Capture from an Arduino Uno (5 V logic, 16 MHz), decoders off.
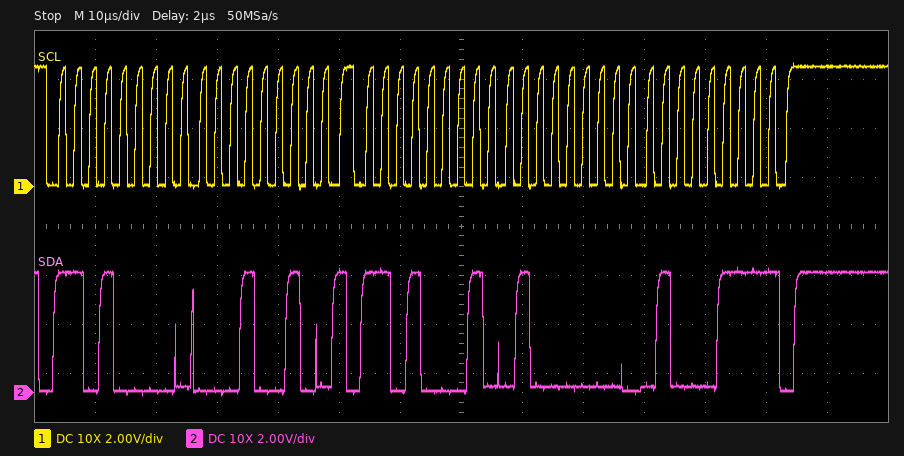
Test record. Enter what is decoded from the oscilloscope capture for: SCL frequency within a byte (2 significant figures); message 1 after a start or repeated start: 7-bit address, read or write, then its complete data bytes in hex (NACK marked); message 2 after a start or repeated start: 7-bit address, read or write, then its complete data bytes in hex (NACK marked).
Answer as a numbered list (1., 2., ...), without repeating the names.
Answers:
1. 400 kHz
2. 0x68 write: 12
3. 0x68 read: 40 47 NACK
